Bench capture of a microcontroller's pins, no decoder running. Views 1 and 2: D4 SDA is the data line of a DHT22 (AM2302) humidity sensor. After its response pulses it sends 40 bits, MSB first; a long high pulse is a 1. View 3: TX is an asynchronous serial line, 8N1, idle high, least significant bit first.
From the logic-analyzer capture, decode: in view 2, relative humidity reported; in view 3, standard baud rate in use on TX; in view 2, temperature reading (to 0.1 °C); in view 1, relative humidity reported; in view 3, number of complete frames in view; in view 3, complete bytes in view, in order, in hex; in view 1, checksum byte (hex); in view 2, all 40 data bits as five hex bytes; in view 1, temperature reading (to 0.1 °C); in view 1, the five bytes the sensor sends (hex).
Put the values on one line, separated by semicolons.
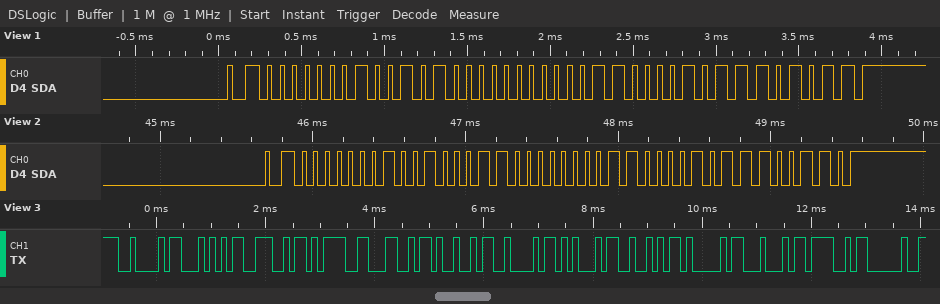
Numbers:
29.1 %; 9600 baud; 19.4 °C; 29.6 %; 13; 42 54 4E 3D 4C 49 42 45 52 41 44 4F 20; 0xEB; 01 23 00 C2 E6; 19.4 °C; 01 28 00 C2 EB
